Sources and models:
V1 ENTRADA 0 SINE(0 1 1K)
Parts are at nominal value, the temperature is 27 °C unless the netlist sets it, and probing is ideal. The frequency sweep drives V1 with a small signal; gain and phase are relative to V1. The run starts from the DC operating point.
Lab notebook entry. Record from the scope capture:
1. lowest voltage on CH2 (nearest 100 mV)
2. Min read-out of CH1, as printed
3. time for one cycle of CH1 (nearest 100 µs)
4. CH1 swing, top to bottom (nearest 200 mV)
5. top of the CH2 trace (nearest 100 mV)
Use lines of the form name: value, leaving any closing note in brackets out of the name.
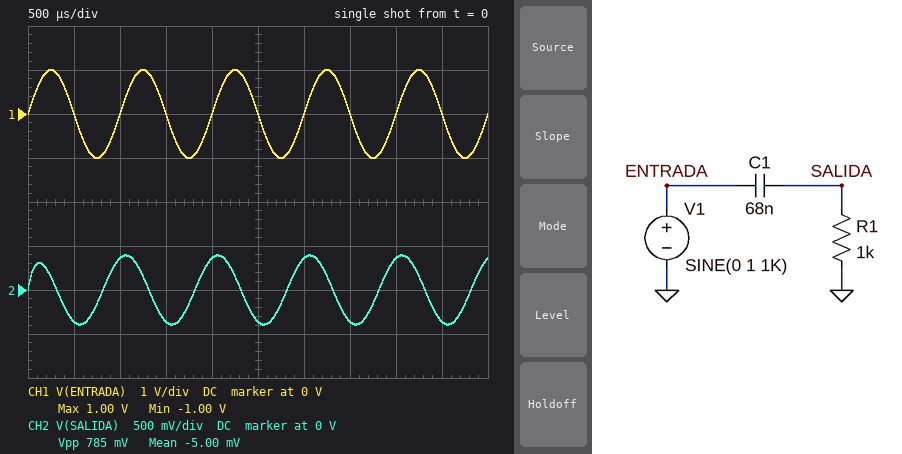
lowest voltage on CH2: -400 mV
Min read-out of CH1, as printed: -1.00 V
time for one cycle of CH1: 1.0 ms
CH1 swing, top to bottom: 2.0 V
top of the CH2 trace: 400 mV
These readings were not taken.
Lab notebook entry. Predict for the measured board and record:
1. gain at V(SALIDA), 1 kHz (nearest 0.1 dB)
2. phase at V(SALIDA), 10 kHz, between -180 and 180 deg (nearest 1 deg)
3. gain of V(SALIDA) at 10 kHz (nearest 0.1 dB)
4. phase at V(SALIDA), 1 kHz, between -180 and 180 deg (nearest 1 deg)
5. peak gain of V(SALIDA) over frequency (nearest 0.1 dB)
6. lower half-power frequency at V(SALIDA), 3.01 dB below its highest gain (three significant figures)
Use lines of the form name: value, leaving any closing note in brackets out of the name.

gain at V(SALIDA), 1 kHz: -8.1 dB
phase at V(SALIDA), 10 kHz, between -180 and 180 deg: 13 deg
gain of V(SALIDA) at 10 kHz: -0.2 dB
phase at V(SALIDA), 1 kHz, between -180 and 180 deg: 67 deg
peak gain of V(SALIDA) over frequency: 0 dB
lower half-power frequency at V(SALIDA), 3.01 dB below its highest gain: 2.34 kHz
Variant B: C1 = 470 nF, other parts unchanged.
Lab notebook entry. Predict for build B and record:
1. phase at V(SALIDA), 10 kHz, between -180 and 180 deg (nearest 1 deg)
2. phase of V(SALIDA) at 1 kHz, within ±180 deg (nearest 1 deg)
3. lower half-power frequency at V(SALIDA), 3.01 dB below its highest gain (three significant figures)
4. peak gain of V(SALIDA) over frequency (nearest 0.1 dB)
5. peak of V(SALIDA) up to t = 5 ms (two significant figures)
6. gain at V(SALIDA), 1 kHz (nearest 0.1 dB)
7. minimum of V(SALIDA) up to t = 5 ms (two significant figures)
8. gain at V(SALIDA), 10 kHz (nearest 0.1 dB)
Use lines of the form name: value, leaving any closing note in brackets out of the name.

phase at V(SALIDA), 10 kHz, between -180 and 180 deg: 2 deg
phase of V(SALIDA) at 1 kHz, within ±180 deg: 19 deg
lower half-power frequency at V(SALIDA), 3.01 dB below its highest gain: 339 Hz
peak gain of V(SALIDA) over frequency: 0 dB
peak of V(SALIDA) up to t = 5 ms: 950 mV
gain at V(SALIDA), 1 kHz: -0.5 dB
minimum of V(SALIDA) up to t = 5 ms: -1.0 V
gain at V(SALIDA), 10 kHz: 0 dB
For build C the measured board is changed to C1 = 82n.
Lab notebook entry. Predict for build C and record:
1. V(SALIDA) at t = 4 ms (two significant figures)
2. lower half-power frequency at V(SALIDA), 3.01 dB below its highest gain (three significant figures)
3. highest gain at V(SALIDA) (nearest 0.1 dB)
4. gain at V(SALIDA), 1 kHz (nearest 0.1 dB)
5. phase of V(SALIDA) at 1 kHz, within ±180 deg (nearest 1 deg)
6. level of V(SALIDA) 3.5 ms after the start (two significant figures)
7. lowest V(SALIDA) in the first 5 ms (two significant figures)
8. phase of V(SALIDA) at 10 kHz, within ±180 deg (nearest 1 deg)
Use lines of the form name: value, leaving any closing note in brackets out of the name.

V(SALIDA) at t = 4 ms: 410 mV
lower half-power frequency at V(SALIDA), 3.01 dB below its highest gain: 1.94 kHz
highest gain at V(SALIDA): 0 dB
gain at V(SALIDA), 1 kHz: -6.8 dB
phase of V(SALIDA) at 1 kHz, within ±180 deg: 63 deg
level of V(SALIDA) 3.5 ms after the start: -410 mV
lowest V(SALIDA) in the first 5 ms: -460 mV
phase of V(SALIDA) at 10 kHz, within ±180 deg: 11 deg
